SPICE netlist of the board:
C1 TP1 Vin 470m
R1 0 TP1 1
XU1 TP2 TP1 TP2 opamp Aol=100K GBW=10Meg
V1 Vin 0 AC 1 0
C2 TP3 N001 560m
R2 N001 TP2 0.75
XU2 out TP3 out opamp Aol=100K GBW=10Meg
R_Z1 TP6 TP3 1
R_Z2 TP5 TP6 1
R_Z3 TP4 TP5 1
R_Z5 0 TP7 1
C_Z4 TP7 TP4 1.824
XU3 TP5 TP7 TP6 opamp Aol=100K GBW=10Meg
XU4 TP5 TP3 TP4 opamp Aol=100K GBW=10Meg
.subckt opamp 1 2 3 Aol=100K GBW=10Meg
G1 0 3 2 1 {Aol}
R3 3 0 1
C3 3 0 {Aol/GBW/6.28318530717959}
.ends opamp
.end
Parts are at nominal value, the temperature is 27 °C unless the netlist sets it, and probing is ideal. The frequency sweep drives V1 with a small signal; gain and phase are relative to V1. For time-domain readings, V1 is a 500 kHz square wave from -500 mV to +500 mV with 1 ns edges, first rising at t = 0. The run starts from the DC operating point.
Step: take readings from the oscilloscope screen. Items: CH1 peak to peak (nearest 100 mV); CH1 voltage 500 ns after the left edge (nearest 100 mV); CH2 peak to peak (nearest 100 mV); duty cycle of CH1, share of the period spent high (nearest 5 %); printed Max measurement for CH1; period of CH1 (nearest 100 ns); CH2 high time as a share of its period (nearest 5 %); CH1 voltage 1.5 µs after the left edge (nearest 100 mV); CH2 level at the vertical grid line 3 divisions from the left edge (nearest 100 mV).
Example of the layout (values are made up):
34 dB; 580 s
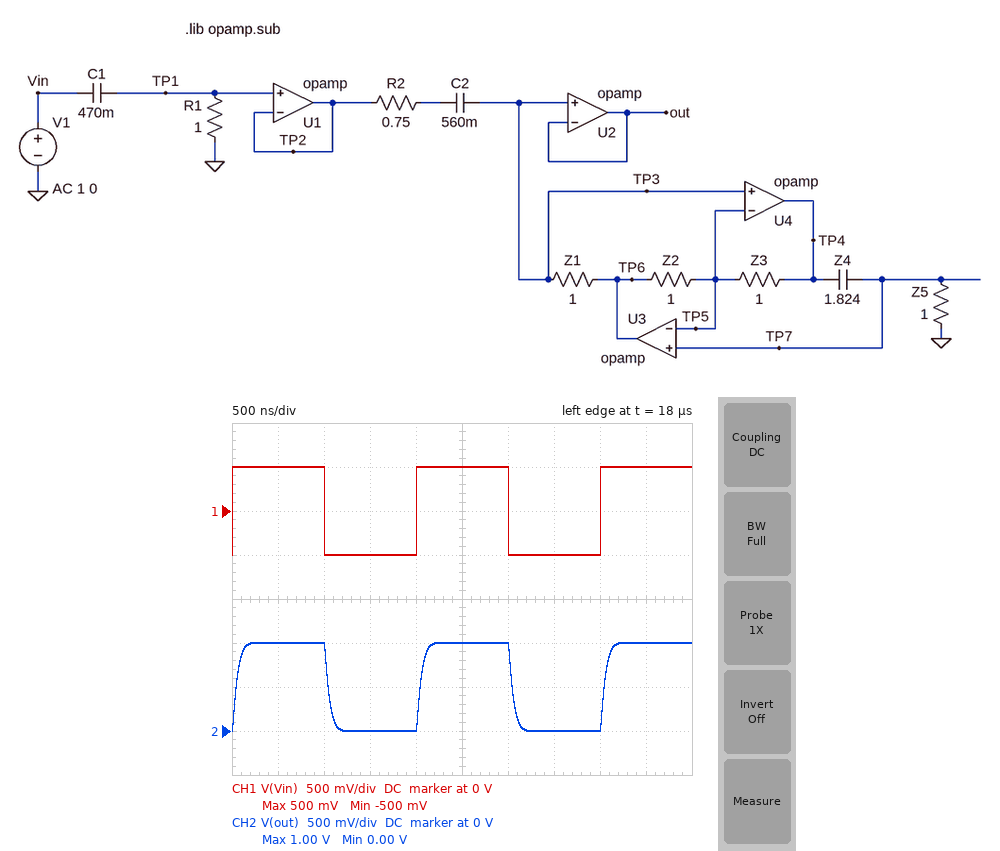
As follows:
1.0 V; 500 mV; 1.0 V; 50 %; 500 mV; 2.0 µs; 50 %; -500 mV; 0 V
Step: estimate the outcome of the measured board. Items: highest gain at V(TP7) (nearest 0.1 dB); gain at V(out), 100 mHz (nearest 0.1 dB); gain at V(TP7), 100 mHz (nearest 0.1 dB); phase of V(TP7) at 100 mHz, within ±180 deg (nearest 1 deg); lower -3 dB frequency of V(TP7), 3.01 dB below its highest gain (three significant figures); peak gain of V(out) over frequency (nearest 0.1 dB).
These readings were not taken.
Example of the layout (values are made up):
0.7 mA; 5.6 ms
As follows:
0.8 dB; -15.1 dB; -15.1 dB; -130 deg; 143 mHz; 0.8 dB
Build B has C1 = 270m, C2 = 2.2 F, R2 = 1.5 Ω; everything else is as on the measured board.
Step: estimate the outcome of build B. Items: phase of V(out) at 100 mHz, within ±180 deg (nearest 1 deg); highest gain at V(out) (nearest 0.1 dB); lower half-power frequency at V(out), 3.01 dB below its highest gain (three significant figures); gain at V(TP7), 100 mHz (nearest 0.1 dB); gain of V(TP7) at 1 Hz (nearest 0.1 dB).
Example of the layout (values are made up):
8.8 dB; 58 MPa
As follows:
155 deg; 0 dB; 597 mHz; -18.2 dB; -1.3 dB
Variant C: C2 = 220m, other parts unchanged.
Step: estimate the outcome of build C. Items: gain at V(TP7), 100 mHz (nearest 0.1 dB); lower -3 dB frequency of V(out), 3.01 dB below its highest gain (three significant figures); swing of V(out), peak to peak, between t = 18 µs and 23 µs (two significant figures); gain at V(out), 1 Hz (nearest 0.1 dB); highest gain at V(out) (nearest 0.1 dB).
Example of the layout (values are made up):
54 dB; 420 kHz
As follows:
-25.5 dB; 231 mHz; 1.0 V; 0.1 dB; 7.4 dB
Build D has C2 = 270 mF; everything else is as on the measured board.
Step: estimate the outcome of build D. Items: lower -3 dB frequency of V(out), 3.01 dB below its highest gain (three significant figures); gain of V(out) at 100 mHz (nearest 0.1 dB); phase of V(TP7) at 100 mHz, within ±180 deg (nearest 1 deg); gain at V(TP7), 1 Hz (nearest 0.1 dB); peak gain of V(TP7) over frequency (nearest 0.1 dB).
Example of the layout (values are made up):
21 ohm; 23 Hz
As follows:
207 mHz; -23.4 dB; -115 deg; 0 dB; 6.0 dB
